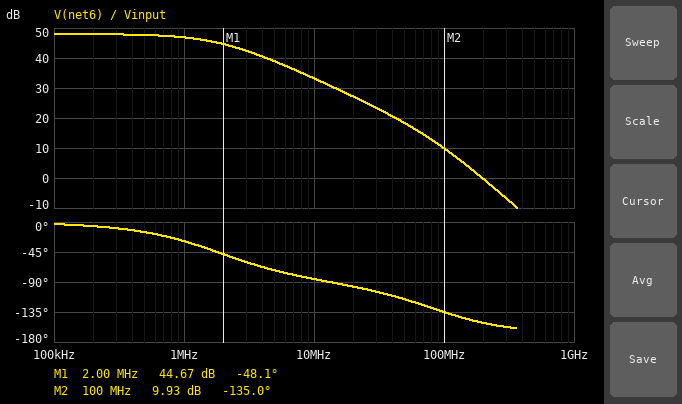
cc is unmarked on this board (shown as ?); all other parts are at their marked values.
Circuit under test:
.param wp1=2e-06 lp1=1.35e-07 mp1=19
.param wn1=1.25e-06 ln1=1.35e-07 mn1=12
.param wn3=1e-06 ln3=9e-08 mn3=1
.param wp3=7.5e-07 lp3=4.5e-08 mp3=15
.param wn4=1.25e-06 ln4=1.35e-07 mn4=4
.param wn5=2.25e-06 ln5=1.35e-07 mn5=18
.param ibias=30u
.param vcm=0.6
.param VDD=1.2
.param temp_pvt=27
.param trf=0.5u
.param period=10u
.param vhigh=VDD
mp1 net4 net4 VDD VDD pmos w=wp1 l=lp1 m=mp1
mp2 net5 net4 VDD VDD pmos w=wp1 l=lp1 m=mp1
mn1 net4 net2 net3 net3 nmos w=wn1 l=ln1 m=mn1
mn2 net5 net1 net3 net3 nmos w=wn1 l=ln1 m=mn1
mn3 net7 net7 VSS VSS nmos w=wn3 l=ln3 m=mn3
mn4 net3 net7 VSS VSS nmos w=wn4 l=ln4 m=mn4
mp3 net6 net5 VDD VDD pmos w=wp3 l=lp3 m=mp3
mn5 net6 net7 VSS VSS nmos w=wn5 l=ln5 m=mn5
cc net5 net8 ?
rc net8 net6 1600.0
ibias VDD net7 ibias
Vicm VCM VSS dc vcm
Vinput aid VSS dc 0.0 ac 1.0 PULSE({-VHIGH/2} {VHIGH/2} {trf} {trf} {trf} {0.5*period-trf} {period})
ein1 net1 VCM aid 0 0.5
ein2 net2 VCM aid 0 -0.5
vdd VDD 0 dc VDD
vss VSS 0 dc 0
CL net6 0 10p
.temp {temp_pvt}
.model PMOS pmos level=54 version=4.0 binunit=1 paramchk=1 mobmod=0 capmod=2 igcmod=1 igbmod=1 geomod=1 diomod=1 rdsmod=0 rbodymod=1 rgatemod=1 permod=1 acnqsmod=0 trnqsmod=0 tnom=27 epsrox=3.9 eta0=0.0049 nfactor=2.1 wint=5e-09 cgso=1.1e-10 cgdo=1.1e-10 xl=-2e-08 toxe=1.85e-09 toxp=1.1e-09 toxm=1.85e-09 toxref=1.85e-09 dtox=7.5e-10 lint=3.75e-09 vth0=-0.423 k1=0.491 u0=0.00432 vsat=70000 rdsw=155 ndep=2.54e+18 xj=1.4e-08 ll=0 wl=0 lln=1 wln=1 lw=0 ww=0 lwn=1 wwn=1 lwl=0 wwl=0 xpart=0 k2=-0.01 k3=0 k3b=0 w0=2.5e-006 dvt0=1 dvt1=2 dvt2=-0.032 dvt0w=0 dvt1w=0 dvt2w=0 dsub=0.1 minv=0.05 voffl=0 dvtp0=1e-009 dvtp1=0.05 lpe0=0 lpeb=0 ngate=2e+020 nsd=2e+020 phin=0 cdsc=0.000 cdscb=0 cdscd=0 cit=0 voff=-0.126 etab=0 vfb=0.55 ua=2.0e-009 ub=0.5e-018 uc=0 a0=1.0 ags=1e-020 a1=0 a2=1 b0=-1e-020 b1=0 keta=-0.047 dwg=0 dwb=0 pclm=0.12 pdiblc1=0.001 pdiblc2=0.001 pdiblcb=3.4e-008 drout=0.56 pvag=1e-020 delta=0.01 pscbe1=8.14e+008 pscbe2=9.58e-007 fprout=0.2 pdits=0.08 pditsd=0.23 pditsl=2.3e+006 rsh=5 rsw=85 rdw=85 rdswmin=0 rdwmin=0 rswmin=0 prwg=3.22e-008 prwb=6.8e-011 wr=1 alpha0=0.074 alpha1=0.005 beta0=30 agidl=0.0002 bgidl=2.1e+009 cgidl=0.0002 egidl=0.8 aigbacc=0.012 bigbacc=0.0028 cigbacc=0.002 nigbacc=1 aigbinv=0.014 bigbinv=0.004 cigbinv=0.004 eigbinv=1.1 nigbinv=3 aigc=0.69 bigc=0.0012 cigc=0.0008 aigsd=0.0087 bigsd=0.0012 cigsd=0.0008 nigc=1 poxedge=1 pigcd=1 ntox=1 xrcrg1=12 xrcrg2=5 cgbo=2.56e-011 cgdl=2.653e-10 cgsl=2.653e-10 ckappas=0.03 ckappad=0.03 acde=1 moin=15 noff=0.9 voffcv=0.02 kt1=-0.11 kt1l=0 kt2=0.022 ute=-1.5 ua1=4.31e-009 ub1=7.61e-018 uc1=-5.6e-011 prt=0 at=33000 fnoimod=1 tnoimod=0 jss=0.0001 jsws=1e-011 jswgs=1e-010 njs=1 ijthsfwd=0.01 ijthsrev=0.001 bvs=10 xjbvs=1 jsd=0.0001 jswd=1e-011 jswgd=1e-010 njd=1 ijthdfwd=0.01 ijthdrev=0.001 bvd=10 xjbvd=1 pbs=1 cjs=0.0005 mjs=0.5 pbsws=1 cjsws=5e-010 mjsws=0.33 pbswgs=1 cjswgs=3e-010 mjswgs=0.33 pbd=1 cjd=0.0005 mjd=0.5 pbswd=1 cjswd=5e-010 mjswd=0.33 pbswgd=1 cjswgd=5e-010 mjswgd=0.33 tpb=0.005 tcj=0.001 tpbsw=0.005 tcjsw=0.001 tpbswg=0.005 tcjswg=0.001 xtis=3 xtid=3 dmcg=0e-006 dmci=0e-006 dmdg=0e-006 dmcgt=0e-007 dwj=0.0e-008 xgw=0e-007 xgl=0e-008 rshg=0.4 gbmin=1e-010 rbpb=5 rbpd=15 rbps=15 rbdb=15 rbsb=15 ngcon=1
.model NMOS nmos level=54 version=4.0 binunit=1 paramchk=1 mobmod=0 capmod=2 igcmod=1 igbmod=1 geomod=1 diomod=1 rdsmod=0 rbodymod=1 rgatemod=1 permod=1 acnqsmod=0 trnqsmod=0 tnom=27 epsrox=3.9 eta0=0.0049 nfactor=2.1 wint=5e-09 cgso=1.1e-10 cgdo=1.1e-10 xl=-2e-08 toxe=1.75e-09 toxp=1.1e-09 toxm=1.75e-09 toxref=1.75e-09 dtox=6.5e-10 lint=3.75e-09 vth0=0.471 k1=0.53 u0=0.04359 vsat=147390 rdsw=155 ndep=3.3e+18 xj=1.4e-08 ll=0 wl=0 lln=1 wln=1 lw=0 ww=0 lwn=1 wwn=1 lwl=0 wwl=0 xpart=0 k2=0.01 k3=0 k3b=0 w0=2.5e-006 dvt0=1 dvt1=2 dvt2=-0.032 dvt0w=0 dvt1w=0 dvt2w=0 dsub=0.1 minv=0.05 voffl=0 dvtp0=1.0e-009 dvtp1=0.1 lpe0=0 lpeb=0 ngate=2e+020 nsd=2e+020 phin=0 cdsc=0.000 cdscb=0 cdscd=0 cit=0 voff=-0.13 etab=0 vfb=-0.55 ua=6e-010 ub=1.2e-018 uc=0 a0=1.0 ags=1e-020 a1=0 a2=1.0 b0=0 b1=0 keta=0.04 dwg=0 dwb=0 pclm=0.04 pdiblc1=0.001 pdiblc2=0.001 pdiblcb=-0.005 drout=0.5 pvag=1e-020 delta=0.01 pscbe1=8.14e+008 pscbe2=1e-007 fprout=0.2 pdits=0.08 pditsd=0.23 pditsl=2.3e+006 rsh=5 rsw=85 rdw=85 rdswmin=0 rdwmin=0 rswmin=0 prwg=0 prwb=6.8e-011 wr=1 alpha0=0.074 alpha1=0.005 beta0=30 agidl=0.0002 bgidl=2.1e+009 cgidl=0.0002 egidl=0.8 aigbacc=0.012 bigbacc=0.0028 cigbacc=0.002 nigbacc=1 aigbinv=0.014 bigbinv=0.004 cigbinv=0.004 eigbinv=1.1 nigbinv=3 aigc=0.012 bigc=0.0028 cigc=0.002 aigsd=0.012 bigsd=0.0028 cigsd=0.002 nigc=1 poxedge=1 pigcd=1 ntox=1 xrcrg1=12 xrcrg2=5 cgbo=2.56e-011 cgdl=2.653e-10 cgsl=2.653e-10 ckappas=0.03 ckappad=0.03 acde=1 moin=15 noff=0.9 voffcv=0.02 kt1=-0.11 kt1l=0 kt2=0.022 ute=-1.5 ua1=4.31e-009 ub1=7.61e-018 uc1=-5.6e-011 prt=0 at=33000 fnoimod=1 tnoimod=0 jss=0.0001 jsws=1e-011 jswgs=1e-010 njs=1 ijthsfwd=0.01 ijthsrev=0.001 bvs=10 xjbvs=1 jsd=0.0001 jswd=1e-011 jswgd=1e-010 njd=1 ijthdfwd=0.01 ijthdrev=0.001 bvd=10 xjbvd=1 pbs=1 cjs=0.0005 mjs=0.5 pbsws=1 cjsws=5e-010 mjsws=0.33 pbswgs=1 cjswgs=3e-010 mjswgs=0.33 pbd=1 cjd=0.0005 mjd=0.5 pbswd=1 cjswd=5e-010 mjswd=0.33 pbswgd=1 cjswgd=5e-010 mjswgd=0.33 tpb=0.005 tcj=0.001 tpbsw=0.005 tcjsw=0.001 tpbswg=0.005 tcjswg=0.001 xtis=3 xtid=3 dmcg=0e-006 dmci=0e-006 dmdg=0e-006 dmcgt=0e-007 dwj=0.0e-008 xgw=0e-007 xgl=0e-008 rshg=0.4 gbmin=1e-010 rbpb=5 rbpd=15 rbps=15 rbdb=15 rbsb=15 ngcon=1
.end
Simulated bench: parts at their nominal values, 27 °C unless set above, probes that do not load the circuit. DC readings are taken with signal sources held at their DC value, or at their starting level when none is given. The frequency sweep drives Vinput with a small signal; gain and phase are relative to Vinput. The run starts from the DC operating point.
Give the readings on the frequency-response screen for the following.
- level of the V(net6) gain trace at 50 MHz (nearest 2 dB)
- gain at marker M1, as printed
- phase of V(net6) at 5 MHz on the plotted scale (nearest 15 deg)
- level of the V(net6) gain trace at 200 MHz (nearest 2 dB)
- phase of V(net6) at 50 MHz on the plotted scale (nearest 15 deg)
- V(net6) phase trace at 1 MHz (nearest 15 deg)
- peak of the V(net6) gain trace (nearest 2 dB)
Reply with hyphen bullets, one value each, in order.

- 18 dB
- 44.67 dB
- -75 deg
- 0 dB
- -120 deg
- -30 deg
- 48 dB
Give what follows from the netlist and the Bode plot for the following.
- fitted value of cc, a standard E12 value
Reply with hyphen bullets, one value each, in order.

- 180 fF
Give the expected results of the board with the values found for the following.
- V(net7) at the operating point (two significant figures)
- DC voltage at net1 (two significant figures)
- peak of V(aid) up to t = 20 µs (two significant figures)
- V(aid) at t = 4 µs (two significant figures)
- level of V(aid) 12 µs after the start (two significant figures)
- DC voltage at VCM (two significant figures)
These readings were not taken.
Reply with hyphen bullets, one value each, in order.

- 520 mV
- 600 mV
- 600 mV
- 600 mV
- 600 mV
- 600 mV
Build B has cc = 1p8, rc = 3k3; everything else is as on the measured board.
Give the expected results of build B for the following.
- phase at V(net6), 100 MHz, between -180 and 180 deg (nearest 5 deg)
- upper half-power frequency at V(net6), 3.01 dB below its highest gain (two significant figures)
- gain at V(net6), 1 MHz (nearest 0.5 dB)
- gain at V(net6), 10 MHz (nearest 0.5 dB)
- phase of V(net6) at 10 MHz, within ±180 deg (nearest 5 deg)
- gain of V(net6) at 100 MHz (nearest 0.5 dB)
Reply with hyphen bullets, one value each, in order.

- -70 deg
- 210 kHz
- 34.5 dB
- 15.0 dB
- -75 deg
- 3.0 dB
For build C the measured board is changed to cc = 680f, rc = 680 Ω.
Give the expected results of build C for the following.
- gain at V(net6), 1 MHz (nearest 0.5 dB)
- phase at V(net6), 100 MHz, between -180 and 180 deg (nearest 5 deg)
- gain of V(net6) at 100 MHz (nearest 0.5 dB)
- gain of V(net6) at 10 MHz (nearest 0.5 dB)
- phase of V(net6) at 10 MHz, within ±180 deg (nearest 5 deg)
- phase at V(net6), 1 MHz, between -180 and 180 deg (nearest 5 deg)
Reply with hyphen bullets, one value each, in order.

- 41.5 dB
- -130 deg
- 0 dB
- 23.0 dB
- -90 deg
- -60 deg
